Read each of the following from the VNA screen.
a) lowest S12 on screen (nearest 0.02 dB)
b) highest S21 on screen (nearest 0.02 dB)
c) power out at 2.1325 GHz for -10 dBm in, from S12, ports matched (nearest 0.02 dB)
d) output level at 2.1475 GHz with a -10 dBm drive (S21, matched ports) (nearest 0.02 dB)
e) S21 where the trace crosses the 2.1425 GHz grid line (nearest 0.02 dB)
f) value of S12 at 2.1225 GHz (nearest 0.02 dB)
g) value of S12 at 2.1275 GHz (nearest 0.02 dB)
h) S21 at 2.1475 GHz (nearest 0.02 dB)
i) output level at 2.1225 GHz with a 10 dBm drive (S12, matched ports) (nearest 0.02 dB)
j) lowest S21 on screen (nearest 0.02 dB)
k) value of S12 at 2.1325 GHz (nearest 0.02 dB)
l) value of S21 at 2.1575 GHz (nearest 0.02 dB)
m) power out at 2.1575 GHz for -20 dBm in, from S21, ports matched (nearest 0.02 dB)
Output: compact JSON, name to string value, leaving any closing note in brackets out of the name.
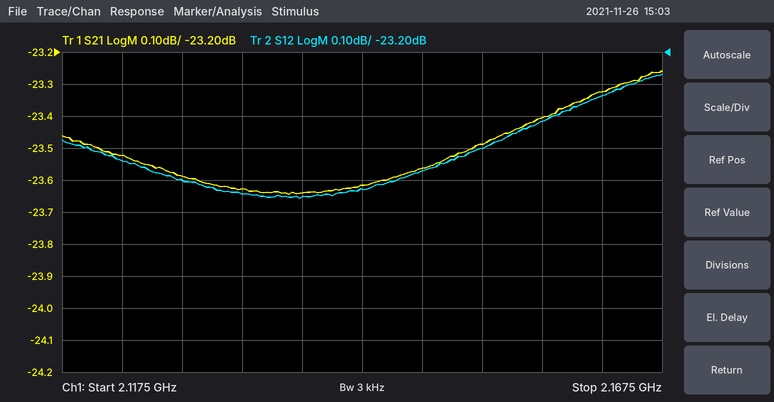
{"lowest S12 on screen": "-23.66 dB", "highest S21 on screen": "-23.26 dB", "power out at 2.1325 GHz for -10 dBm in, from S12, ports matched": "-33.64 dBm", "output level at 2.1475 GHz with a -10 dBm drive (S21, matched ports)": "-33.56 dBm", "S21 where the trace crosses the 2.1425 GHz grid line": "-23.62 dB", "value of S12 at 2.1225 GHz": "-23.54 dB", "value of S12 at 2.1275 GHz": "-23.60 dB", "S21 at 2.1475 GHz": "-23.56 dB", "output level at 2.1225 GHz with a 10 dBm drive (S12, matched ports)": "-13.54 dBm", "lowest S21 on screen": "-23.64 dB", "value of S12 at 2.1325 GHz": "-23.64 dB", "value of S21 at 2.1575 GHz": "-23.40 dB", "power out at 2.1575 GHz for -20 dBm in, from S21, ports matched": "-43.40 dBm"}
